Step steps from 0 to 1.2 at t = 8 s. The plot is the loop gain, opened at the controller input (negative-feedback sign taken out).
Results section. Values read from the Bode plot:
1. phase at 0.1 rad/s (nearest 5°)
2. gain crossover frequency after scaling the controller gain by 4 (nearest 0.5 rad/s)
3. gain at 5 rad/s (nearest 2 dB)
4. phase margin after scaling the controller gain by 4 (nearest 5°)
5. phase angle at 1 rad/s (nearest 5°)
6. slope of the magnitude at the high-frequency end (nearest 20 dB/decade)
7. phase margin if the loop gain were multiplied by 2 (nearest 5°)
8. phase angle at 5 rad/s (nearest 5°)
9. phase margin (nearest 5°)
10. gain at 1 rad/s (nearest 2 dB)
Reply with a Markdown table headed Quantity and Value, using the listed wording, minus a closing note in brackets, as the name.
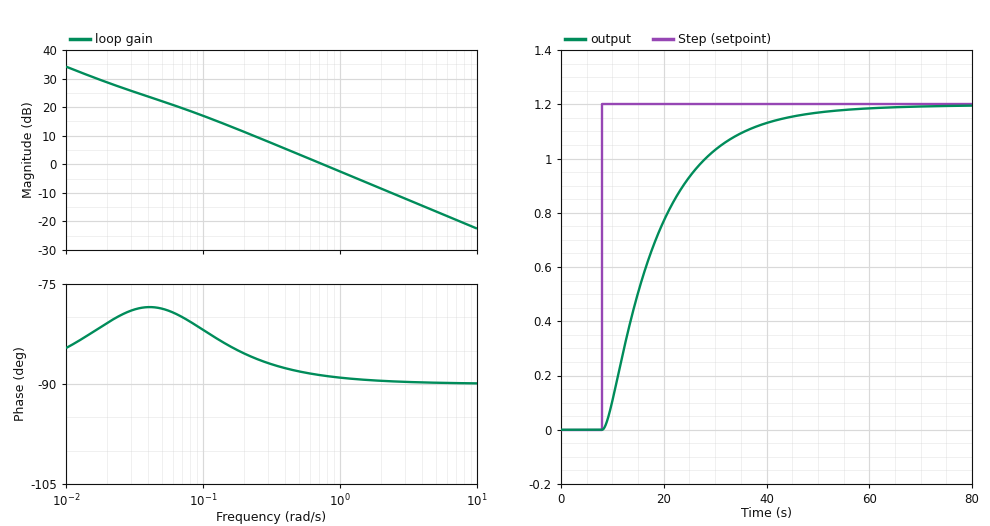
| Quantity | Value |
|---|---|
| phase at 0.1 rad/s | -80° |
| gain crossover frequency after scaling the controller gain by 4 | 3.0 rad/s |
| gain at 5 rad/s | -16 dB |
| phase margin after scaling the controller gain by 4 | 90° |
| phase angle at 1 rad/s | -90° |
| slope of the magnitude at the high-frequency end | -20 dB/decade |
| phase margin if the loop gain were multiplied by 2 | 90° |
| phase angle at 5 rad/s | -90° |
| phase margin | 90° |
| gain at 1 rad/s | -2 dB |
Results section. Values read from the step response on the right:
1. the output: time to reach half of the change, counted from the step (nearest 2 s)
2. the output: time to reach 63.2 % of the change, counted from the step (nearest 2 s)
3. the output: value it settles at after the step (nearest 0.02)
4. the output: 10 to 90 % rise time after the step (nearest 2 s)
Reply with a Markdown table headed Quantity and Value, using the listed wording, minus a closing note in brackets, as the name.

| Quantity | Value |
|---|---|
| the output: time to reach half of the change, counted from the step | 8 s |
| the output: time to reach 63.2 % of the change, counted from the step | 12 s |
| the output: value it settles at after the step | 1.20 |
| the output: 10 to 90 % rise time after the step | 24 s |
